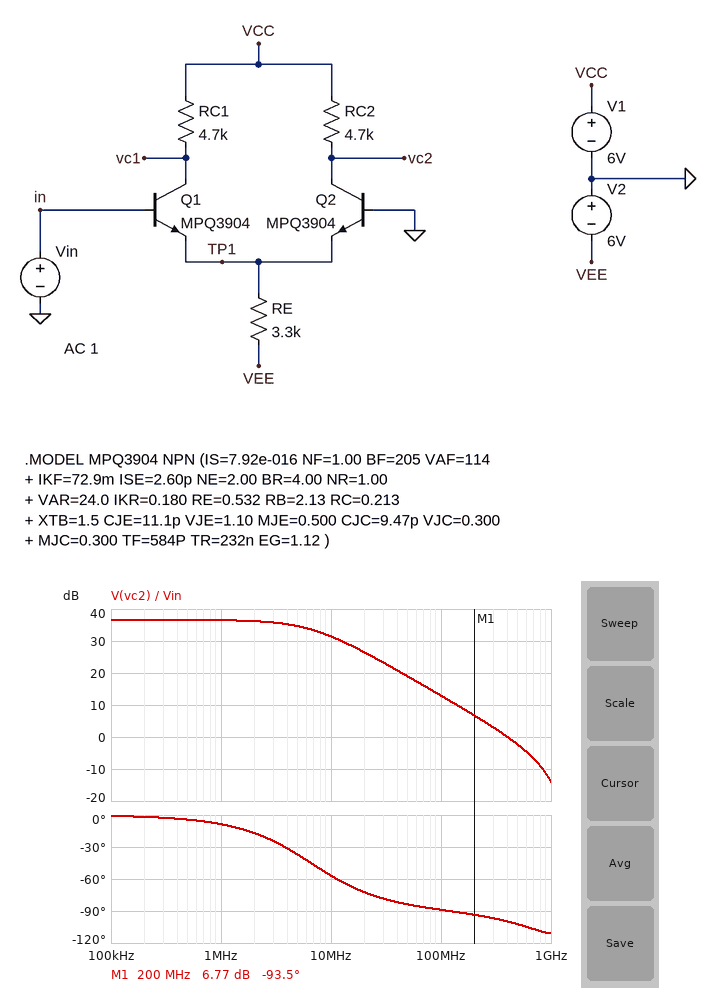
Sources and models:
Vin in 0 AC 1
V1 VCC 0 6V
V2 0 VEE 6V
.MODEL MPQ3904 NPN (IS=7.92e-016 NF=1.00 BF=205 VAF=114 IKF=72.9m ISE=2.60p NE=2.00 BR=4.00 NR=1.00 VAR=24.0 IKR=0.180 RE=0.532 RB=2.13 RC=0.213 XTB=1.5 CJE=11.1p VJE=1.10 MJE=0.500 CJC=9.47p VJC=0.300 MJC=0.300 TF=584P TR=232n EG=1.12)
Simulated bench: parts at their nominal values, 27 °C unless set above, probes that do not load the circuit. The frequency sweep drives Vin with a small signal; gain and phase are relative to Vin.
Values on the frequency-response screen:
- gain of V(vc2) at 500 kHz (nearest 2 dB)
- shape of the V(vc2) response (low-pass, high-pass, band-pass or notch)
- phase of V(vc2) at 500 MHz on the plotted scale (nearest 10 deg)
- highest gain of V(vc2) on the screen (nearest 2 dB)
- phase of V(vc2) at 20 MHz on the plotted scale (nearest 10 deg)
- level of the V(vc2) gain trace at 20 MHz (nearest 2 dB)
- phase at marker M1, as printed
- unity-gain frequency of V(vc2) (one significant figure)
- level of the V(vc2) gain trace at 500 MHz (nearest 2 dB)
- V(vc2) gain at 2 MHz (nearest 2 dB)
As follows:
36 dB
low-pass
-100 deg
36 dB
-70 deg
26 dB
-93.5 deg
400 MHz
-2 dB
36 dB
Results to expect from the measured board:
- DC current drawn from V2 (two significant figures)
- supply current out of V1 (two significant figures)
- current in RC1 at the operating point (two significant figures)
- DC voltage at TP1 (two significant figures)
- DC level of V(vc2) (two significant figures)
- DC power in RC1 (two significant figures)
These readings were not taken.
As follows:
1.6 mA
1.6 mA
790 µA
-720 mV
2.3 V
3.0 mW
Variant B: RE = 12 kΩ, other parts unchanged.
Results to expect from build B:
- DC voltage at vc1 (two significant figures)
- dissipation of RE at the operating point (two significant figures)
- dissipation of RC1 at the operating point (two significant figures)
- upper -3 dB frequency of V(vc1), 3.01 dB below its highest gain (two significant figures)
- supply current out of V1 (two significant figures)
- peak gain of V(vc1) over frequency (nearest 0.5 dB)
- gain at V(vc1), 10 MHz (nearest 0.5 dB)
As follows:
5.0 V
2.4 mW
230 µW
8.4 MHz
440 µA
26.0 dB
22.0 dB
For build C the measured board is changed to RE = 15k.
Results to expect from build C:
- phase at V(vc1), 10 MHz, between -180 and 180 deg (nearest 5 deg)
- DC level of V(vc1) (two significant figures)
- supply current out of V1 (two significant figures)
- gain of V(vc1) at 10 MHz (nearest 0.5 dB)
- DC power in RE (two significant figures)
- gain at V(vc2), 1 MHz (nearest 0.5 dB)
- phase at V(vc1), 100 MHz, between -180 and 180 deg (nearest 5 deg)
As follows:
125 deg
5.2 V
350 µA
20.0 dB
1.9 mW
24.0 dB
55 deg
